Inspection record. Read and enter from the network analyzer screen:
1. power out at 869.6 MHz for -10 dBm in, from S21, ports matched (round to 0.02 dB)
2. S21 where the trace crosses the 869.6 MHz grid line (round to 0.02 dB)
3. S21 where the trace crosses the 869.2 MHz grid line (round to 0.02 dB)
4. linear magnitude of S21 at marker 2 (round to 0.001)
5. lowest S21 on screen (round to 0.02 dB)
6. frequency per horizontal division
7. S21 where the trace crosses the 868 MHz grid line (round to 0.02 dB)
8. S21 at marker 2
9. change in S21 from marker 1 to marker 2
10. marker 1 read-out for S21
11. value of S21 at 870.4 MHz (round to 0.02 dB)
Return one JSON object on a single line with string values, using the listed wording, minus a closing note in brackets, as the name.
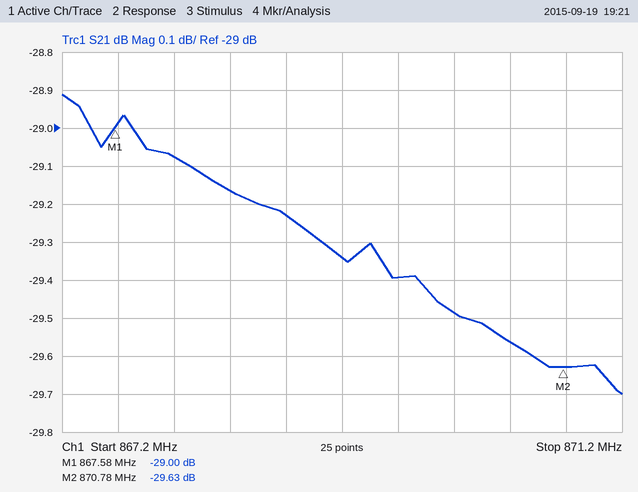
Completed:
{"power out at 869.6 MHz for -10 dBm in, from S21, ports matched": "-39.40 dBm", "S21 where the trace crosses the 869.6 MHz grid line": "-29.40 dB", "S21 where the trace crosses the 869.2 MHz grid line": "-29.34 dB", "linear magnitude of S21 at marker 2": "0.033", "lowest S21 on screen": "-29.70 dB", "frequency per horizontal division": "400 kHz", "S21 where the trace crosses the 868 MHz grid line": "-29.08 dB", "S21 at marker 2": "-29.63 dB", "change in S21 from marker 1 to marker 2": "-0.63 dB", "marker 1 read-out for S21": "-29.00 dB", "value of S21 at 870.4 MHz": "-29.56 dB"}
